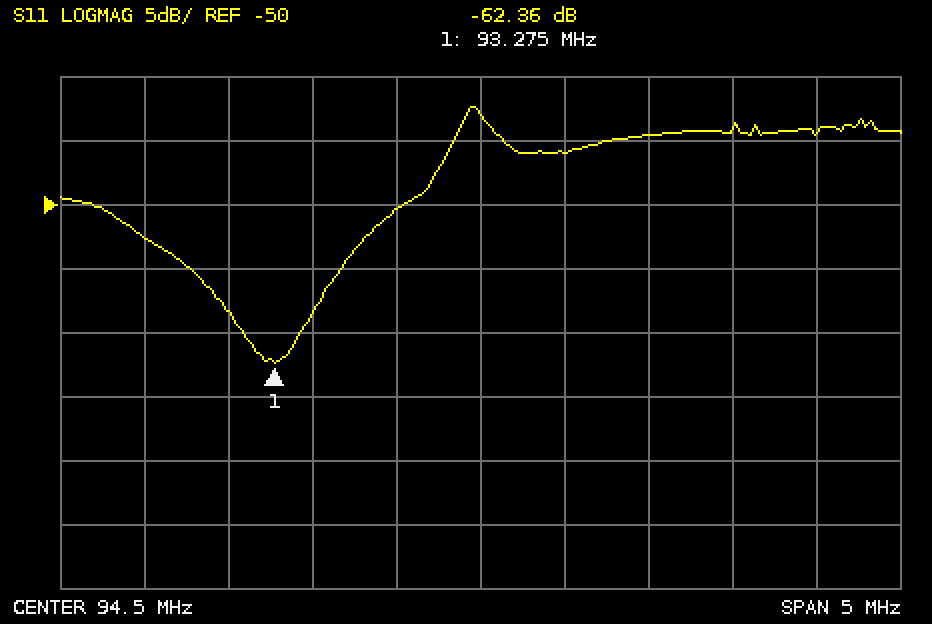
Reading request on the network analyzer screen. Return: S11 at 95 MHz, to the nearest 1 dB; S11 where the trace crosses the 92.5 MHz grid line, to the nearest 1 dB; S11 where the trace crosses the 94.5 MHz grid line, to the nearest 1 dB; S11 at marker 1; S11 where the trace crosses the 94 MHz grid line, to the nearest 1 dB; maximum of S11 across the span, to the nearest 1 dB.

-46 dB
-53 dB
-43 dB
-62.36 dB
-50 dB
-42 dB
